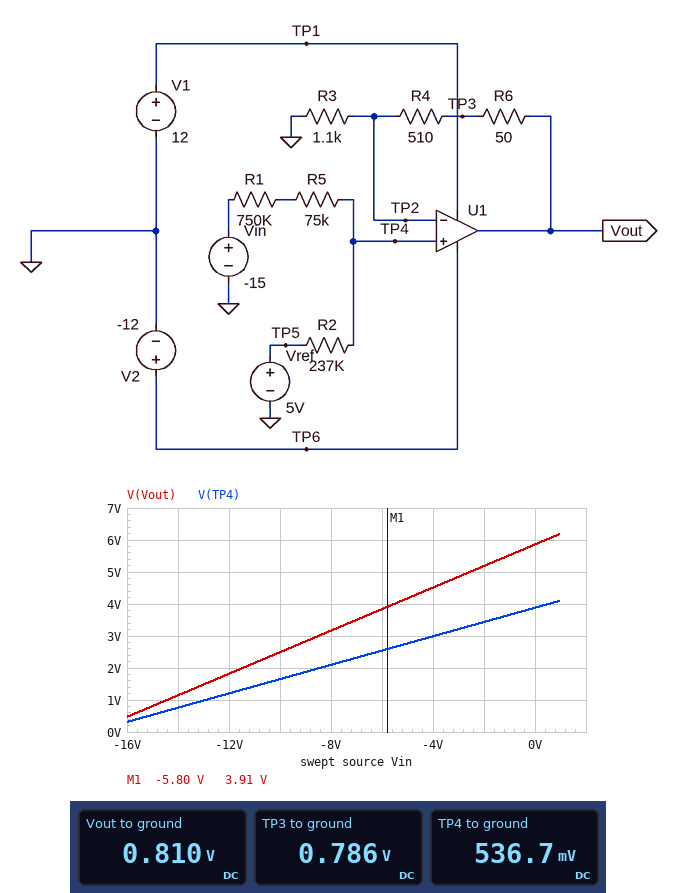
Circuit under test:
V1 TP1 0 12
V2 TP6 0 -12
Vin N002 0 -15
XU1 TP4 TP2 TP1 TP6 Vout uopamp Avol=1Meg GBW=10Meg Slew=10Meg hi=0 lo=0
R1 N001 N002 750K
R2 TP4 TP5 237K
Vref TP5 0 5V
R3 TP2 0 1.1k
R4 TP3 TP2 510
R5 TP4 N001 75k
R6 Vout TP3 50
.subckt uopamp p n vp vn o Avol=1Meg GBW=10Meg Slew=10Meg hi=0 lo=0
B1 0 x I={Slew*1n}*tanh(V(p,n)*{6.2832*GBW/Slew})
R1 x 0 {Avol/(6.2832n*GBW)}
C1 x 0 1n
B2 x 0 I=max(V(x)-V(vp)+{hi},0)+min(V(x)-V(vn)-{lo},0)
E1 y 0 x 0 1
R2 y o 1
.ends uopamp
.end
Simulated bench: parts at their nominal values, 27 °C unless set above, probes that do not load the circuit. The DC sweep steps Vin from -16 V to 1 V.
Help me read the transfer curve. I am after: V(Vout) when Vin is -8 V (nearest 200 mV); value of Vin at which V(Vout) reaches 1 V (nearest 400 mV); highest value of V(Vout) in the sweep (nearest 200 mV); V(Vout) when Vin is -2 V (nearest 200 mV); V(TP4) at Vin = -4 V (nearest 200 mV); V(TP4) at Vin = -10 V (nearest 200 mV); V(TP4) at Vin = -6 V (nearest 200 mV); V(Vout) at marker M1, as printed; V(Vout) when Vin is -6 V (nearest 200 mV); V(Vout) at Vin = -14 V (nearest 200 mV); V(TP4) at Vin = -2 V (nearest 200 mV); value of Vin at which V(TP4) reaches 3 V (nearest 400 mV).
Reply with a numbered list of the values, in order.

1. 3.2 V
2. -14.4 V
3. 6.2 V
4. 5.2 V
5. 3.0 V
6. 1.6 V
7. 2.6 V
8. 3.91 V
9. 3.8 V
10. 1.2 V
11. 3.4 V
12. -4.0 V
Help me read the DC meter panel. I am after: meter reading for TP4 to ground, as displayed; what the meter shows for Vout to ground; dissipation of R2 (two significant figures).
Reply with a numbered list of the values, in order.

1. 536.7 mV
2. 0.810 V
3. 84 µW
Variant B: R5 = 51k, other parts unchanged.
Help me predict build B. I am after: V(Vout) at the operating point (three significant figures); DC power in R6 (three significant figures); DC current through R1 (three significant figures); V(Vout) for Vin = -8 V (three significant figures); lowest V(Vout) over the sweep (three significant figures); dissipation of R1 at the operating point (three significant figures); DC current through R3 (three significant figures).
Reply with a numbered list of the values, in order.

1. 654 mV
2. 7.77 µW
3. 19.3 µA
4. 3.07 V
5. 310 mV
6. 278 µW
7. 394 µA
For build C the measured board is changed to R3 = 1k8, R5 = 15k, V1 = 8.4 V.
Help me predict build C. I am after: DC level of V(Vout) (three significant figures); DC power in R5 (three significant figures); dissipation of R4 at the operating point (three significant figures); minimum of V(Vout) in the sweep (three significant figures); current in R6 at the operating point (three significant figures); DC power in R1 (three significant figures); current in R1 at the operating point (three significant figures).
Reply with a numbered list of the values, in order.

1. 353 mV
2. 5.98 µW
3. 11.4 µW
4. 43.2 mV
5. 150 µA
6. 299 µW
7. 20.0 µA
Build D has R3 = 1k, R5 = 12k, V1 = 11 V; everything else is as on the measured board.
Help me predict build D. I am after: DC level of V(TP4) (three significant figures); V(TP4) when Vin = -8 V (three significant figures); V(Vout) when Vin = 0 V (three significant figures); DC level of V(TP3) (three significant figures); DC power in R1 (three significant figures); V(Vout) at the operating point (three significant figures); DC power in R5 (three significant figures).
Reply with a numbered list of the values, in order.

1. 255 mV
2. 1.92 V
3. 5.95 V
4. 385 mV
5. 301 µW
6. 398 mV
7. 4.81 µW
